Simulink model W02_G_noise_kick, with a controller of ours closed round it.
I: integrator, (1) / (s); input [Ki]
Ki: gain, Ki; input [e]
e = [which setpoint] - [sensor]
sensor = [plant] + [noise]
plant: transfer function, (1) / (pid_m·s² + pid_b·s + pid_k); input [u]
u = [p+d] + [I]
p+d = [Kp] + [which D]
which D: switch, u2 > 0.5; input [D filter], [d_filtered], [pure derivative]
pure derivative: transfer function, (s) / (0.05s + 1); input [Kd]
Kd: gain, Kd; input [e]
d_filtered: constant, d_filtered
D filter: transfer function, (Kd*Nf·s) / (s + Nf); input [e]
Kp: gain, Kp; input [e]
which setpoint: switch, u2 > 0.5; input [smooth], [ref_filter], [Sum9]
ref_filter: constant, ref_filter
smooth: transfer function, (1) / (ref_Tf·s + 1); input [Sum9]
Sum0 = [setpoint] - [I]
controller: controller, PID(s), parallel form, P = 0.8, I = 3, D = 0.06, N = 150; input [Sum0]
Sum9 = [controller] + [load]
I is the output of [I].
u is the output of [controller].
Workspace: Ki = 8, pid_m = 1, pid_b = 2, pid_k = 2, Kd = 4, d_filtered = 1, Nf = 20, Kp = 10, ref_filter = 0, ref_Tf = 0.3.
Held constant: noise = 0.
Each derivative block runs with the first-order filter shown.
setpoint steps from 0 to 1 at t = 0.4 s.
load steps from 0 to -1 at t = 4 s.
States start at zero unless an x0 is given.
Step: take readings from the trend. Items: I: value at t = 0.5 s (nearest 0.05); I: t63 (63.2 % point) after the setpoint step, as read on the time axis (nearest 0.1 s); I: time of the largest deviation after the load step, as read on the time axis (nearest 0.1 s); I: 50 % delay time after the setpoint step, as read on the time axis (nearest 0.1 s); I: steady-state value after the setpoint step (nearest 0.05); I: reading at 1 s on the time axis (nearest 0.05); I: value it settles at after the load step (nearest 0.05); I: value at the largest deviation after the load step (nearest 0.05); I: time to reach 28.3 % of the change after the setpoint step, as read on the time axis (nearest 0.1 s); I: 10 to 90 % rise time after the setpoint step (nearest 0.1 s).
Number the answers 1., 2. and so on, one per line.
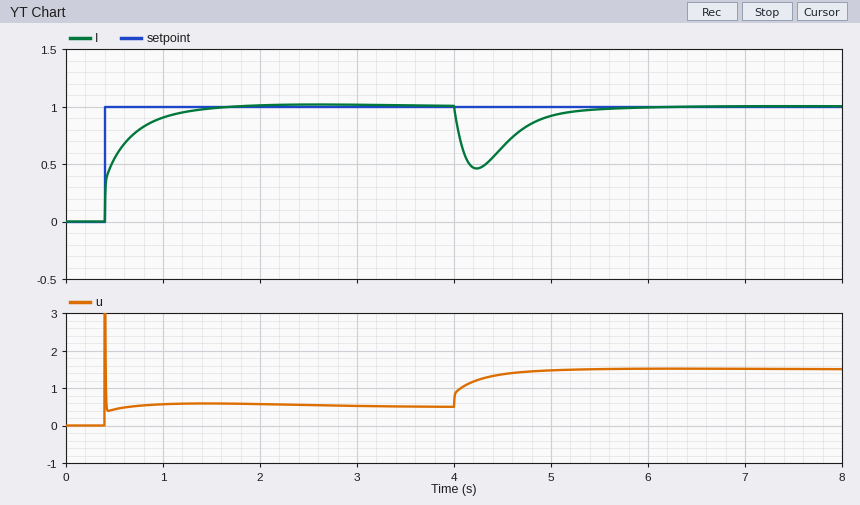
1. 0.55
2. 0.6 s
3. 4.2 s
4. 0.5 s
5. 1.00
6. 0.90
7. 1.00
8. 0.45
9. 0.4 s
10. 0.6 s
